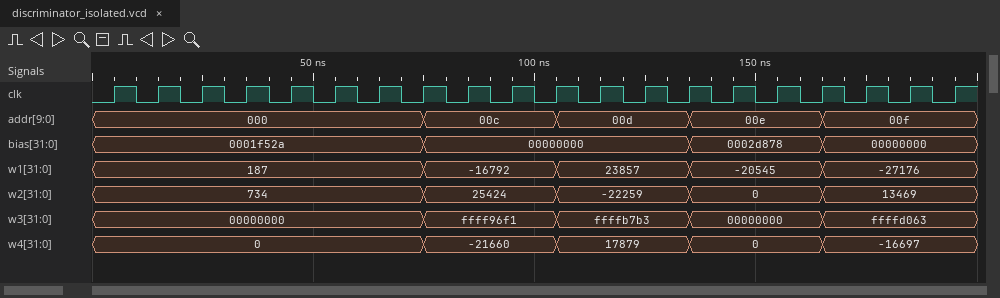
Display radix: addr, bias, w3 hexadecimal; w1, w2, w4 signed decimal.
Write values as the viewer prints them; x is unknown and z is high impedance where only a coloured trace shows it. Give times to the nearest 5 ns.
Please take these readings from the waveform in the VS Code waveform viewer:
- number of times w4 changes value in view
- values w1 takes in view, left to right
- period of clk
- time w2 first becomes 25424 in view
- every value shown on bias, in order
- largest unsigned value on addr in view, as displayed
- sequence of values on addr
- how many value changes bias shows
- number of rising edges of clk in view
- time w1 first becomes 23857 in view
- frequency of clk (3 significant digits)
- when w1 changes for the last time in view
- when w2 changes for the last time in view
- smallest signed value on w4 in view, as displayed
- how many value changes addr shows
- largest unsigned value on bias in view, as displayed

4
187, -16792, 23857, -20545, -27176
10 ns
75 ns
0001f52a, 00000000, 0002d878, 00000000
00f
000, 00c, 00d, 00e, 00f
3
20
105 ns
100 MHz
165 ns
165 ns
-21660
4
0002d878
